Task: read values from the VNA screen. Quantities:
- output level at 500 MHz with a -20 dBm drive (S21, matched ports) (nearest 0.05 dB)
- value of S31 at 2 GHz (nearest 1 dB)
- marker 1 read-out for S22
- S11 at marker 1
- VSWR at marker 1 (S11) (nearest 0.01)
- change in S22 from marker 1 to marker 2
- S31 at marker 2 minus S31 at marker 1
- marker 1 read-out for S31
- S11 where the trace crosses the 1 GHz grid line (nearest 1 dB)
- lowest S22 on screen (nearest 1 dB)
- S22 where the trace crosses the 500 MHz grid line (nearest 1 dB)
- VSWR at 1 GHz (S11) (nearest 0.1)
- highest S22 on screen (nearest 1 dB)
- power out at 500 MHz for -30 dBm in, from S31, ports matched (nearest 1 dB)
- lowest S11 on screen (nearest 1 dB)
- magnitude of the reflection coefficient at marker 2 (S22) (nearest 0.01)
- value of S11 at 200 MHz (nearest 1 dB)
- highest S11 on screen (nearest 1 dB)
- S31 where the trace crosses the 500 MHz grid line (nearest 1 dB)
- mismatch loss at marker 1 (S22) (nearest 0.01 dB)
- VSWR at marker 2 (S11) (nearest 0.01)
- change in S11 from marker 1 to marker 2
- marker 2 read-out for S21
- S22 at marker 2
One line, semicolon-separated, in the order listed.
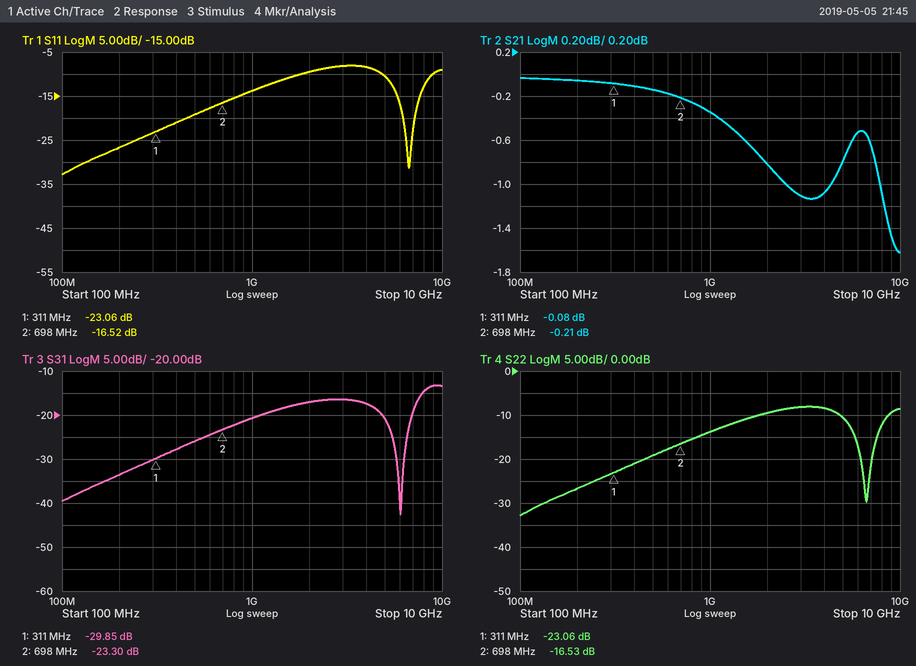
-20.15 dBm; -17 dB; -23.06 dB; -23.06 dB; 1.15; 6.53 dB; 6.55 dB; -29.85 dB; -14 dB; -33 dB; -19 dB; 1.5; -8 dB; -56 dBm; -33 dB; 0.15; -27 dB; -8 dB; -26 dB; 0.02 dB; 1.35; 6.54 dB; -0.21 dB; -16.53 dB
